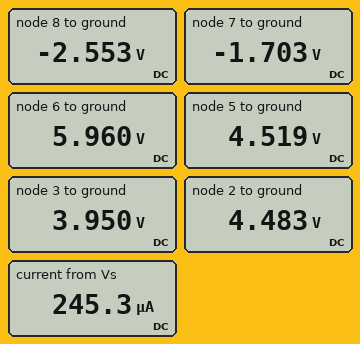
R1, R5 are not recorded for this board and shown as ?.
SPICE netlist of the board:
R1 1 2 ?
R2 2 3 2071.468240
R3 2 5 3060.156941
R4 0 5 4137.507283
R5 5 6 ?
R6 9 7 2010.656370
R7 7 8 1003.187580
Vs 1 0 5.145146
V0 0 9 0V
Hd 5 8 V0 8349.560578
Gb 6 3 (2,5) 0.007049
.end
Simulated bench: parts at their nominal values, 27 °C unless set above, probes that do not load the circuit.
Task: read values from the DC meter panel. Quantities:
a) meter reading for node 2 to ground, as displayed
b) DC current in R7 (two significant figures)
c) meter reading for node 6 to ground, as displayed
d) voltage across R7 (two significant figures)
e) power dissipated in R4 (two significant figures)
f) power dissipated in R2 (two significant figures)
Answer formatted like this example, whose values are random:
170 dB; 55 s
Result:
4.483 V; 850 µA; 5.960 V; 850 mV; 4.9 mW; 140 µW
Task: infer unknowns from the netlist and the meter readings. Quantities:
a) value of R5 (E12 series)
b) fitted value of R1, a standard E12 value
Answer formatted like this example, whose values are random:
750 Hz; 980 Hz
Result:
5.6 kΩ; 2.7 kΩ
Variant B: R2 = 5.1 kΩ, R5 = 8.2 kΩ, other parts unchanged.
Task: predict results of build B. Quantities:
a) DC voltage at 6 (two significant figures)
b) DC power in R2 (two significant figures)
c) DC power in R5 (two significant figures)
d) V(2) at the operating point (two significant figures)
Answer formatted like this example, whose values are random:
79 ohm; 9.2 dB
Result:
6.6 V; 340 µW; 540 µW; 4.5 V
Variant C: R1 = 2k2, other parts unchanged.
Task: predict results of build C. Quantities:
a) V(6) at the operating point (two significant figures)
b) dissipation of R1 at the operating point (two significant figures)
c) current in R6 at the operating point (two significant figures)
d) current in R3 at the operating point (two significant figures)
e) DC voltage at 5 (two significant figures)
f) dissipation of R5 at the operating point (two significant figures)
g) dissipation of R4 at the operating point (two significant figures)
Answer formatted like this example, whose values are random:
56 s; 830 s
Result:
6.1 V; 140 µW; 870 µA; 12 µA; 4.6 V; 390 µW; 5.2 mW
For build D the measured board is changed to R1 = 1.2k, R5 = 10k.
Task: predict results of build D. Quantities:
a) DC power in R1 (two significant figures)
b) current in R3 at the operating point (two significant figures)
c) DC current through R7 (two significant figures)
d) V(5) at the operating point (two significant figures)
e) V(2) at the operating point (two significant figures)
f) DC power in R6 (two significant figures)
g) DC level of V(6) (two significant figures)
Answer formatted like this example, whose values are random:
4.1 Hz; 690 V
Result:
84 µW; 13 µA; 910 µA; 4.9 V; 4.8 V; 1.7 mW; 7.6 V
